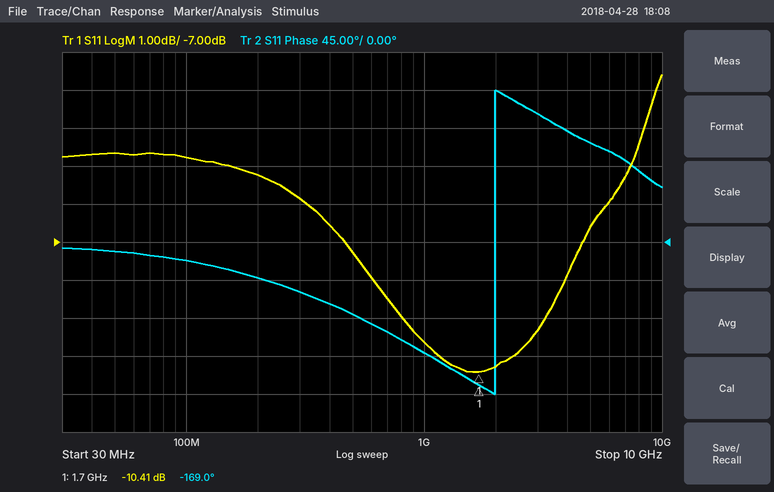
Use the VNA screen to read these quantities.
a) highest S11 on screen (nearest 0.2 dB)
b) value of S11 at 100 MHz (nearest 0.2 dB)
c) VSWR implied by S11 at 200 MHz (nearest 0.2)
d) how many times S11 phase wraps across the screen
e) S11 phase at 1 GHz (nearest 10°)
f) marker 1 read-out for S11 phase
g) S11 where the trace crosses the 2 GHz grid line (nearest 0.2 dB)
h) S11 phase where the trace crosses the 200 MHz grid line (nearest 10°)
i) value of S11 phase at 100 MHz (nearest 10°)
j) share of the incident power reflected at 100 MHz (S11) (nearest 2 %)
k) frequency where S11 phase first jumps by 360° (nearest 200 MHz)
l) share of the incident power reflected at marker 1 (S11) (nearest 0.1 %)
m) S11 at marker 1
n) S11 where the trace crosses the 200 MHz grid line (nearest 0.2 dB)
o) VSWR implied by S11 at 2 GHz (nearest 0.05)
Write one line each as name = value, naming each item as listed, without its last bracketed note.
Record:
highest S11 on screen = -2.6 dB
value of S11 at 100 MHz = -4.8 dB
VSWR implied by S11 at 200 MHz = 3.4
how many times S11 phase wraps across the screen = 1
S11 phase at 1 GHz = -130°
marker 1 read-out for S11 phase = -169.0°
S11 where the trace crosses the 2 GHz grid line = -10.2 dB
S11 phase where the trace crosses the 200 MHz grid line = -40°
value of S11 phase at 100 MHz = -20°
share of the incident power reflected at 100 MHz (S11) = 34 %
frequency where S11 phase first jumps by 360° = 2.0 GHz
share of the incident power reflected at marker 1 (S11) = 9.1 %
S11 at marker 1 = -10.41 dB
S11 where the trace crosses the 200 MHz grid line = -5.2 dB
VSWR implied by S11 at 2 GHz = 1.90
